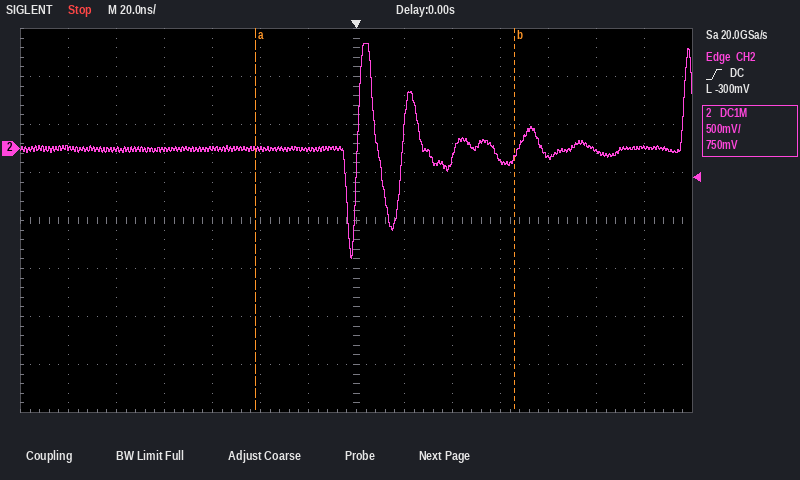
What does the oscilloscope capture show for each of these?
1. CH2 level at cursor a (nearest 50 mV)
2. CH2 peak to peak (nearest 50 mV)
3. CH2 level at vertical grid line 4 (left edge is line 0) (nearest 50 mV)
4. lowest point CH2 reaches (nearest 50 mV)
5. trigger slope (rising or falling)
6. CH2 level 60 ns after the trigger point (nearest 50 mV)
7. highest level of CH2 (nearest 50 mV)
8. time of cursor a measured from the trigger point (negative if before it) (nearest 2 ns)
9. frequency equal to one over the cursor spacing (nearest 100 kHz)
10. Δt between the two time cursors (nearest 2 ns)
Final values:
0 mV
2.25 V
0 mV
-1.15 V
rising
-150 mV
1.10 V
-42 ns
9.3 MHz
108 ns
